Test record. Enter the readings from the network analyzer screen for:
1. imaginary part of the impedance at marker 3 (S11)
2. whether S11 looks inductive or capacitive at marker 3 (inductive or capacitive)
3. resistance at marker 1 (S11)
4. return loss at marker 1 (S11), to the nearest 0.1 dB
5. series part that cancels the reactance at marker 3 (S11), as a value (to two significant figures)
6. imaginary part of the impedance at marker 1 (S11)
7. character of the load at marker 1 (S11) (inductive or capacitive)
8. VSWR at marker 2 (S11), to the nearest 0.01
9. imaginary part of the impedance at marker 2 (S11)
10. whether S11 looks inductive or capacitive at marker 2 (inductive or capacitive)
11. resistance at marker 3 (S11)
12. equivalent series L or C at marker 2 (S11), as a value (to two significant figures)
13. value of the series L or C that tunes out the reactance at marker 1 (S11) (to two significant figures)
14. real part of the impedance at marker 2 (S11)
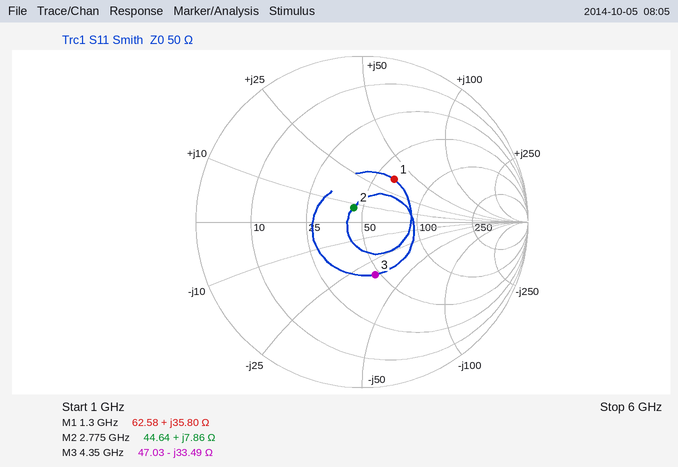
-33.49 Ω
capacitive
62.58 Ω
9.9 dB
1.2 nH
+35.80 Ω
inductive
1.22
+7.86 Ω
inductive
47.03 Ω
450 pH
3.4 pF
44.64 Ω
